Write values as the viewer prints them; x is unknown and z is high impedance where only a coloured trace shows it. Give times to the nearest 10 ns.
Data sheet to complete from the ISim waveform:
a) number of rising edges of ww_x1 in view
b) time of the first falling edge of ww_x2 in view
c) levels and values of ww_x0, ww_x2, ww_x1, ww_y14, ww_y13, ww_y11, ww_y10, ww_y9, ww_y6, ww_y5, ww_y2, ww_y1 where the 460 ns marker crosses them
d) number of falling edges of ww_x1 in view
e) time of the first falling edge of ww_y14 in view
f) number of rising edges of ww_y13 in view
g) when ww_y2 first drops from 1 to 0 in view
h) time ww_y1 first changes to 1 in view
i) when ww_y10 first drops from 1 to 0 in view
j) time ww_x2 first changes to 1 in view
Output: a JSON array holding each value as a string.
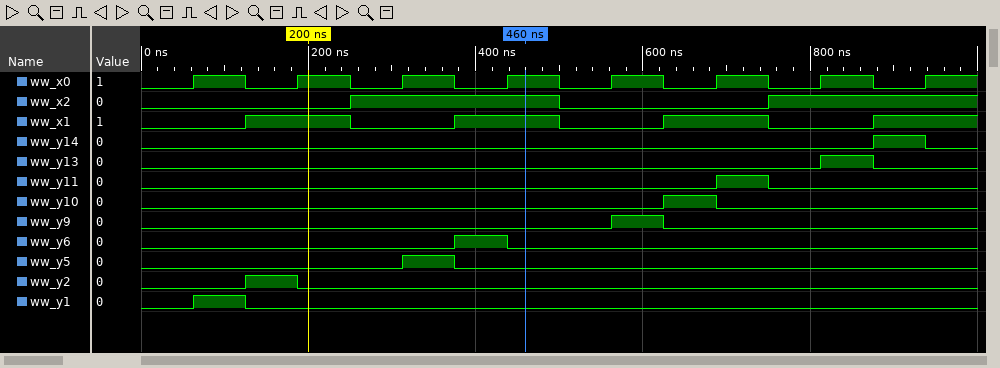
["4", "500 ns", "ww_x0=1, ww_x2=1, ww_x1=1, ww_y14=0, ww_y13=0, ww_y11=0, ww_y10=0, ww_y9=0, ww_y6=0, ww_y5=0, ww_y2=0, ww_y1=0", "3", "940 ns", "1", "190 ns", "60 ns", "690 ns", "250 ns"]
